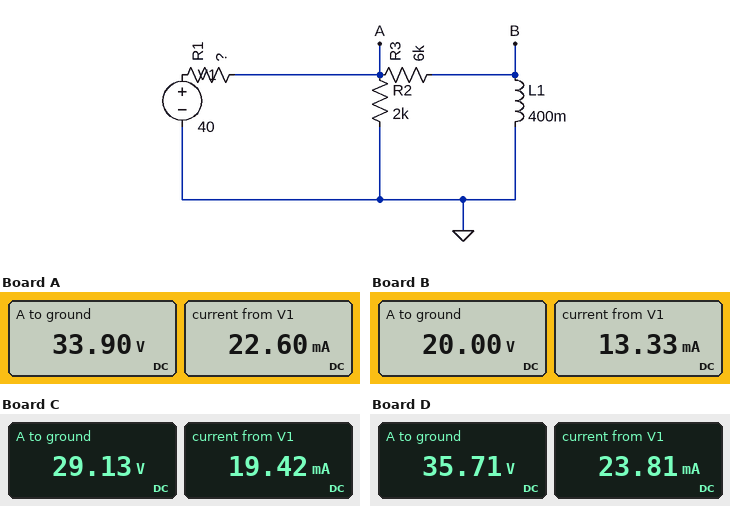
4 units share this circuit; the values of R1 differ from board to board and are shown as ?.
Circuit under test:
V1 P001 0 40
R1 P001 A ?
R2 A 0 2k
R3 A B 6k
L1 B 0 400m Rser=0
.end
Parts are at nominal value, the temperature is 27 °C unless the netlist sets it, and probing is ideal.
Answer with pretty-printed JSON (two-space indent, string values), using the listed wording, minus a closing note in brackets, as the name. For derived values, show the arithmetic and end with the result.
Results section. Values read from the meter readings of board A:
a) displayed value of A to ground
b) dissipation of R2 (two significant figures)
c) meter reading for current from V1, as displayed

{
  "displayed value of A to ground": "33.90 V",
  "dissipation of R2": "(33.9 V)^2 / 2 kΩ = 570 mW",
  "meter reading for current from V1, as displayed": "22.60 mA"
}
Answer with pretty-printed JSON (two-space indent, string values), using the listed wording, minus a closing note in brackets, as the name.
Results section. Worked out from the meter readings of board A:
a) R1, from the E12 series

{
  "R1, from the E12 series": "270 Ω"
}
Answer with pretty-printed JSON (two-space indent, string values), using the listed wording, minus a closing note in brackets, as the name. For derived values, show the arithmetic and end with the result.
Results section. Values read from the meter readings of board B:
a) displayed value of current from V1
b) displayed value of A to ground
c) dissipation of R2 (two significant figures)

{
  "displayed value of current from V1": "13.33 mA",
  "displayed value of A to ground": "20.00 V",
  "dissipation of R2": "(20 V)^2 / 2 kΩ = 200 mW"
}
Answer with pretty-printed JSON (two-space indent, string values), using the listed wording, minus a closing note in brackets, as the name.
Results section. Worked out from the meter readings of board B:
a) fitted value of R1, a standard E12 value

{
  "fitted value of R1, a standard E12 value": "1.5 kΩ"
}
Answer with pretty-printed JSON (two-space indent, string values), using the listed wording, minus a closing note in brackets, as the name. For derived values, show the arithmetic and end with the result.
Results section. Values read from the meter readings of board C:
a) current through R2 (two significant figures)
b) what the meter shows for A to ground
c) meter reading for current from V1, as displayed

{
  "current through R2": "(29.13 V) / 2 kΩ = 15 mA",
  "what the meter shows for A to ground": "29.13 V",
  "meter reading for current from V1, as displayed": "19.42 mA"
}
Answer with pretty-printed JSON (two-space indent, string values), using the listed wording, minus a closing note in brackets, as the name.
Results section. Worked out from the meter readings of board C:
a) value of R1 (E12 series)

{
  "value of R1": "560 Ω"
}
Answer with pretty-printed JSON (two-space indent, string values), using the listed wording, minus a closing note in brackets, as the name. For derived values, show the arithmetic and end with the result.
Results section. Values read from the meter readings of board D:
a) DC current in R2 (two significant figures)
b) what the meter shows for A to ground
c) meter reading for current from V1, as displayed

{
  "DC current in R2": "(35.71 V) / 2 kΩ = 18 mA",
  "what the meter shows for A to ground": "35.71 V",
  "meter reading for current from V1, as displayed": "23.81 mA"
}
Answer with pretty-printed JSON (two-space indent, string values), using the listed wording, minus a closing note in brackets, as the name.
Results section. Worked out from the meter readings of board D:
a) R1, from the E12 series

{
  "R1, from the E12 series": "180 Ω"
}
